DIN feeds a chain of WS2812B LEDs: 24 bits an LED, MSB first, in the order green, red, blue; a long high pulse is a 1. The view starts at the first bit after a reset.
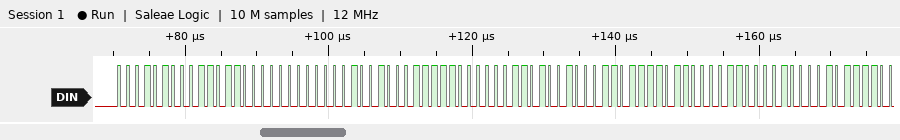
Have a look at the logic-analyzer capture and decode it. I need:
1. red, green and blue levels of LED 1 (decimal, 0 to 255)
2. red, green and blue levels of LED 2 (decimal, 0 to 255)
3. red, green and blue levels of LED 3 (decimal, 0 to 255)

108, 20, 0
124, 36, 13
123, 35, 12
